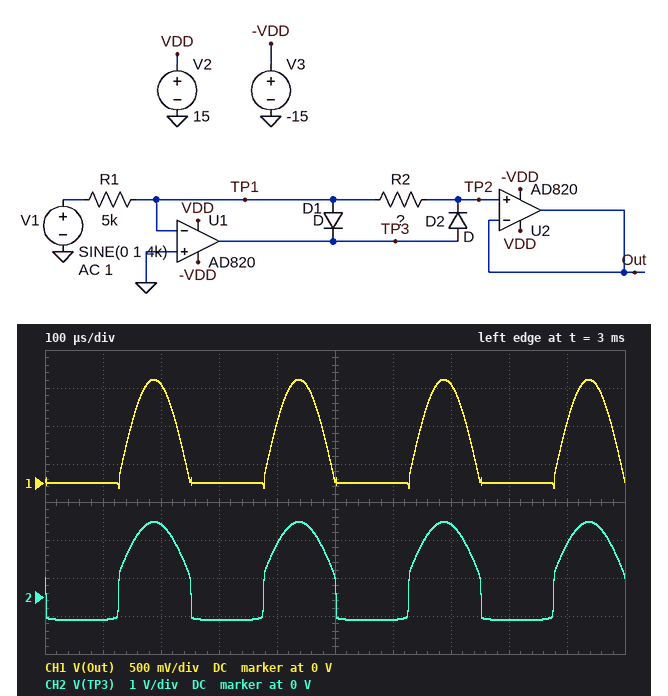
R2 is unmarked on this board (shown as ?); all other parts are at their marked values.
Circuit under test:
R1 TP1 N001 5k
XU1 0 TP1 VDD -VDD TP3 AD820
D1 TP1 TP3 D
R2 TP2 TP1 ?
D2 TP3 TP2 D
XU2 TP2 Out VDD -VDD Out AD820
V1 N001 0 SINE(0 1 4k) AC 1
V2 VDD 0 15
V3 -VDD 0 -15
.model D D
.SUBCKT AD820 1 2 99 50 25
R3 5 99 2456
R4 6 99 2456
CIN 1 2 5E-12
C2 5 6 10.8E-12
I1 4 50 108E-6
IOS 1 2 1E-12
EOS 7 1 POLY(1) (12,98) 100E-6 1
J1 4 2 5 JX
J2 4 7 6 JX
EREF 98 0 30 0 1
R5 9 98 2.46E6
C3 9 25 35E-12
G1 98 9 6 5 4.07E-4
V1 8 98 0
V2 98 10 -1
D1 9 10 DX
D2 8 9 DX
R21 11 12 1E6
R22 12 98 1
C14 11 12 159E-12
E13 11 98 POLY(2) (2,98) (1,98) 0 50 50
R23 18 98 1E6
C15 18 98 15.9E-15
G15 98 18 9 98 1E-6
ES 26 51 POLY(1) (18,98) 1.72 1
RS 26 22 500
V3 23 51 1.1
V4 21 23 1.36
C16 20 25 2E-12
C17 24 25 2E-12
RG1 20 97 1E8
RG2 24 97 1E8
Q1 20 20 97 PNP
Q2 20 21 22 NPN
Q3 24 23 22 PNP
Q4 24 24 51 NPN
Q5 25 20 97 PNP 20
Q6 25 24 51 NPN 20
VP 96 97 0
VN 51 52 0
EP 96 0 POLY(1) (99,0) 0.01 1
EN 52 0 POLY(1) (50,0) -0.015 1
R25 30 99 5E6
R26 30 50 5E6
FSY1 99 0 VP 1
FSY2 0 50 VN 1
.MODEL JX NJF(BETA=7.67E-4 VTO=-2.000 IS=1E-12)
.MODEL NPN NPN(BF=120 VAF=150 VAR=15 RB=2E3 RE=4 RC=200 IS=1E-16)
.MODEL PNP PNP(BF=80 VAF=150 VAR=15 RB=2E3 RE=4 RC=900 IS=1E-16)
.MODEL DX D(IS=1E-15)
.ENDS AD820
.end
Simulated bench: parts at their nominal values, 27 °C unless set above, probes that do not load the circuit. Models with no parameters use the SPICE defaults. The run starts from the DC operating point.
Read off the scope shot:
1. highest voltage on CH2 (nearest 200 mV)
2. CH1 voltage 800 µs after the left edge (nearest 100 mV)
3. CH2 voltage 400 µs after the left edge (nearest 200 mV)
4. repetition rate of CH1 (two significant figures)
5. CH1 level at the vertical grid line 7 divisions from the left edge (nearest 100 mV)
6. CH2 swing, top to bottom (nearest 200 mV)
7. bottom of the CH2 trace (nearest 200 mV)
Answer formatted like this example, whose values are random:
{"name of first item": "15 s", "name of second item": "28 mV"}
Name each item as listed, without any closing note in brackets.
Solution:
{"highest voltage on CH2": "2.0 V", "CH1 voltage 800 µs after the left edge": "0 V", "CH2 voltage 400 µs after the left edge": "1.4 V", "repetition rate of CH1": "4.0 kHz", "CH1 level at the vertical grid line 7 divisions from the left edge": "1.3 V", "CH2 swing, top to bottom": "2.6 V", "bottom of the CH2 trace": "-600 mV"}
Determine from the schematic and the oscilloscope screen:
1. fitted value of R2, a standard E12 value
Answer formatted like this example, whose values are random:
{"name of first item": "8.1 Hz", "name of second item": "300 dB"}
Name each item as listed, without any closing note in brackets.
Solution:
{"fitted value of R2, a standard E12 value": "6.8 kΩ"}
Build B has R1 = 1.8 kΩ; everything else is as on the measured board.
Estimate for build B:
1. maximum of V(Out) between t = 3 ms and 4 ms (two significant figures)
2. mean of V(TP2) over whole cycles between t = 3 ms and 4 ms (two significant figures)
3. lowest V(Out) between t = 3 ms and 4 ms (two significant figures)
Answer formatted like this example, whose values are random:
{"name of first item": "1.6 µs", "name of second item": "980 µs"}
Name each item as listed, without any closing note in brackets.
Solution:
{"maximum of V(Out) between t = 3 ms and 4 ms": "3.8 V", "mean of V(TP2) over whole cycles between t = 3 ms and 4 ms": "1.2 V", "lowest V(Out) between t = 3 ms and 4 ms": "-62 mV"}
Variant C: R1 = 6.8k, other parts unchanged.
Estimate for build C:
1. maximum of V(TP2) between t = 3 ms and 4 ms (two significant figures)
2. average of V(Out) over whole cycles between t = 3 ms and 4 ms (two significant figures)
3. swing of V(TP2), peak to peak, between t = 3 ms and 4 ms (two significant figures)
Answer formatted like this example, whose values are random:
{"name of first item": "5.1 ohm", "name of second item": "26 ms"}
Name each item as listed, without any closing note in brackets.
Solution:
{"maximum of V(TP2) between t = 3 ms and 4 ms": "1.0 V", "average of V(Out) over whole cycles between t = 3 ms and 4 ms": "320 mV", "swing of V(TP2), peak to peak, between t = 3 ms and 4 ms": "1.1 V"}
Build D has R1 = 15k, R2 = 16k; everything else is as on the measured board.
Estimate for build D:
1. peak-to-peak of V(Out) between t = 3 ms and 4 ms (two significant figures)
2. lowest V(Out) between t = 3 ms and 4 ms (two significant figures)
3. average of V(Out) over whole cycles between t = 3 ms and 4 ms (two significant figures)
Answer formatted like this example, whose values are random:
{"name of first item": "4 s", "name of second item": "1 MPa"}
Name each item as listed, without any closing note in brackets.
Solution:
{"peak-to-peak of V(Out) between t = 3 ms and 4 ms": "1.1 V", "lowest V(Out) between t = 3 ms and 4 ms": "-59 mV", "average of V(Out) over whole cycles between t = 3 ms and 4 ms": "340 mV"}
